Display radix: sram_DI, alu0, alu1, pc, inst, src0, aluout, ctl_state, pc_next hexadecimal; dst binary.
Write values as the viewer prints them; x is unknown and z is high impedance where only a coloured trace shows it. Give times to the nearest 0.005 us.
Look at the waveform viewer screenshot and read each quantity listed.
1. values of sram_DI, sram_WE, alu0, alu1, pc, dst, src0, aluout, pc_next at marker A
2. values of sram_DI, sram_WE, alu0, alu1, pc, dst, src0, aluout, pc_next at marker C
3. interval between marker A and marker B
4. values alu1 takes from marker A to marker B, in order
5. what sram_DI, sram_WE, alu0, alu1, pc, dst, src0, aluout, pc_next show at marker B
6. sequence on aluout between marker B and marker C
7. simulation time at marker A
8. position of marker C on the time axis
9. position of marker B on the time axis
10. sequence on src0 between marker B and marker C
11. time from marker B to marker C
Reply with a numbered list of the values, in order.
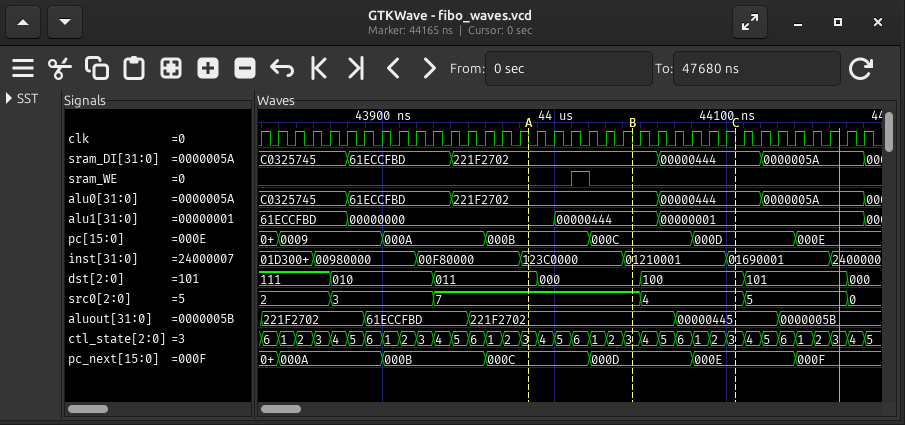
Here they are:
1. sram_DI=221F2702, sram_WE=0, alu0=221F2702, alu1=00000000, pc=000B, dst=011, src0=7, aluout=221F2702, pc_next=000C
2. sram_DI=00000444, sram_WE=0, alu0=00000444, alu1=00000001, pc=000D, dst=100, src0=4, aluout=00000445, pc_next=000E
3. 0.06 us
4. 00000000, 00000444
5. sram_DI=221F2702, sram_WE=0, alu0=221F2702, alu1=00000444, pc=000C, dst=000, src0=7, aluout=221F2702, pc_next=000D
6. 221F2702, 00000445
7. 43.985 us
8. 44.105 us
9. 44.045 us
10. 7, 4
11. 0.06 us
